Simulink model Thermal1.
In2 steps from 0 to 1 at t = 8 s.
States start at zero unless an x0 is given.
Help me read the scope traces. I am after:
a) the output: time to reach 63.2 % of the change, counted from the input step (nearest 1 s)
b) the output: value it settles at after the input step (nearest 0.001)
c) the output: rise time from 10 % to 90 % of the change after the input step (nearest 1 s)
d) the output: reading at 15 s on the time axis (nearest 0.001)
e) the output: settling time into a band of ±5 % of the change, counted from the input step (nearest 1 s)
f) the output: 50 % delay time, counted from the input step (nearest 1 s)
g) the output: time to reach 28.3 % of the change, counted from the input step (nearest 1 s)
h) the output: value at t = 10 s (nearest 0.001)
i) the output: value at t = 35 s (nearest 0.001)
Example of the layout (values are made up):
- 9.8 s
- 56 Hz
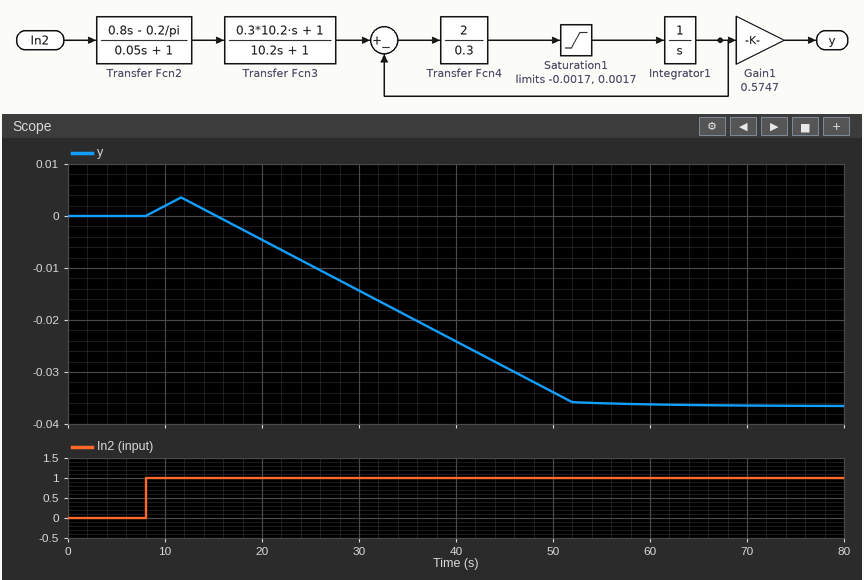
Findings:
- 31 s
- -0.037
- 30 s
- 0.000
- 43 s
- 26 s
- 18 s
- 0.002
- -0.019
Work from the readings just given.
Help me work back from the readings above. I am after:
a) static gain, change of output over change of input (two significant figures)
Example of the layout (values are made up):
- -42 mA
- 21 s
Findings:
- -0.037
